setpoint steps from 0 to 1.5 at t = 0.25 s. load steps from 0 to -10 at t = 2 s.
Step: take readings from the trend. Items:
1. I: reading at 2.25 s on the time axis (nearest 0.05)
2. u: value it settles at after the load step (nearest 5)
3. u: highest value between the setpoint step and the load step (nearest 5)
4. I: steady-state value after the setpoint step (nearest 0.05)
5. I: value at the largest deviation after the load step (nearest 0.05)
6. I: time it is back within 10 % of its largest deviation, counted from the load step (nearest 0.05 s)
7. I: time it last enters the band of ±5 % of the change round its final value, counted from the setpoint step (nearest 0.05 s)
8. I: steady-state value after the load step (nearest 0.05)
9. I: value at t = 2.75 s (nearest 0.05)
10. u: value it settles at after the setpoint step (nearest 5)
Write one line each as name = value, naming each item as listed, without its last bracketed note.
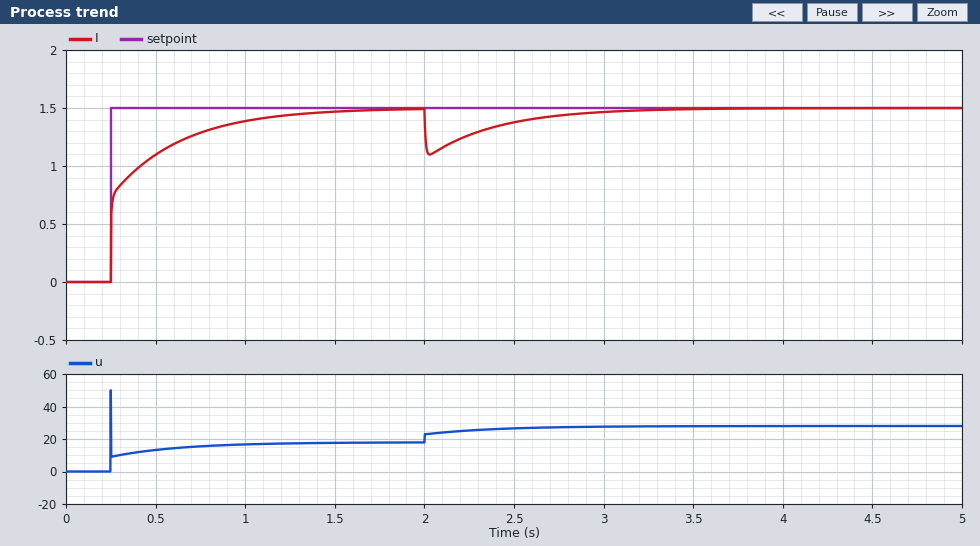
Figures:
I: reading at 2.25 s on the time axis = 1.25
u: value it settles at after the load step = 30
u: highest value between the setpoint step and the load step = 50
I: steady-state value after the setpoint step = 1.50
I: value at the largest deviation after the load step = 1.10
I: time it is back within 10 % of its largest deviation, counted from the load step = 0.95 s
I: time it last enters the band of ±5 % of the change round its final value, counted from the setpoint step = 0.90 s
I: steady-state value after the load step = 1.50
I: value at t = 2.75 s = 1.45
u: value it settles at after the setpoint step = 20
